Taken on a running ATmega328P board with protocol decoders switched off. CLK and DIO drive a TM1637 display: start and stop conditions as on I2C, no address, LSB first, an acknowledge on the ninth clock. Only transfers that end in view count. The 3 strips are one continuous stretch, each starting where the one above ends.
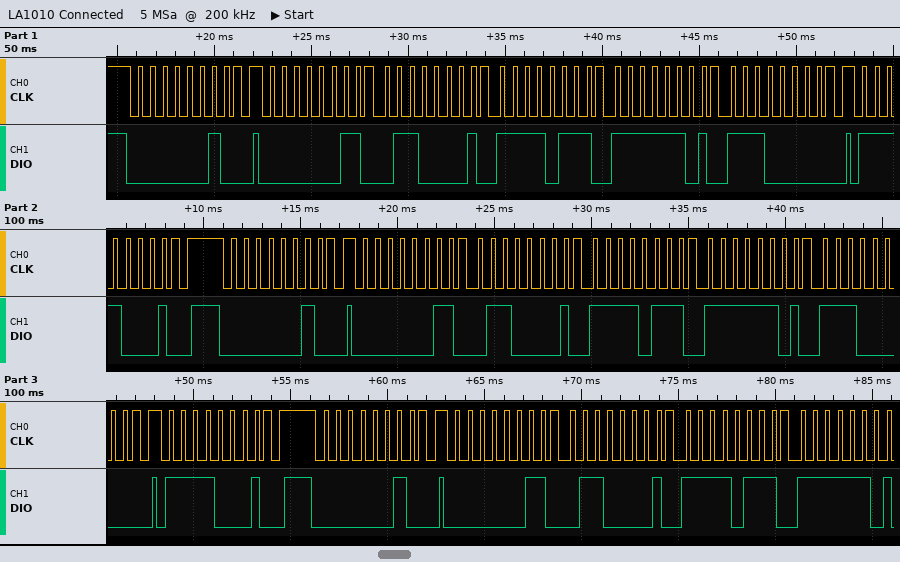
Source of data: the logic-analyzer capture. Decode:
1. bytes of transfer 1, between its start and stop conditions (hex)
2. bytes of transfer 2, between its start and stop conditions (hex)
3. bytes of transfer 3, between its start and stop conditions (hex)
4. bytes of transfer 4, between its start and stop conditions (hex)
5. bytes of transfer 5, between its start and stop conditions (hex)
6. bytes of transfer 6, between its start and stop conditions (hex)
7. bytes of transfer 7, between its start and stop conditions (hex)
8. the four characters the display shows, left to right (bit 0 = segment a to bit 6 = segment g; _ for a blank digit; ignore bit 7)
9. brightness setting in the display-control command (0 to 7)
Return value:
40
C0 86 EF BF 07
8F
40
C0 86 EF BF 07
8F
40
1907
7
